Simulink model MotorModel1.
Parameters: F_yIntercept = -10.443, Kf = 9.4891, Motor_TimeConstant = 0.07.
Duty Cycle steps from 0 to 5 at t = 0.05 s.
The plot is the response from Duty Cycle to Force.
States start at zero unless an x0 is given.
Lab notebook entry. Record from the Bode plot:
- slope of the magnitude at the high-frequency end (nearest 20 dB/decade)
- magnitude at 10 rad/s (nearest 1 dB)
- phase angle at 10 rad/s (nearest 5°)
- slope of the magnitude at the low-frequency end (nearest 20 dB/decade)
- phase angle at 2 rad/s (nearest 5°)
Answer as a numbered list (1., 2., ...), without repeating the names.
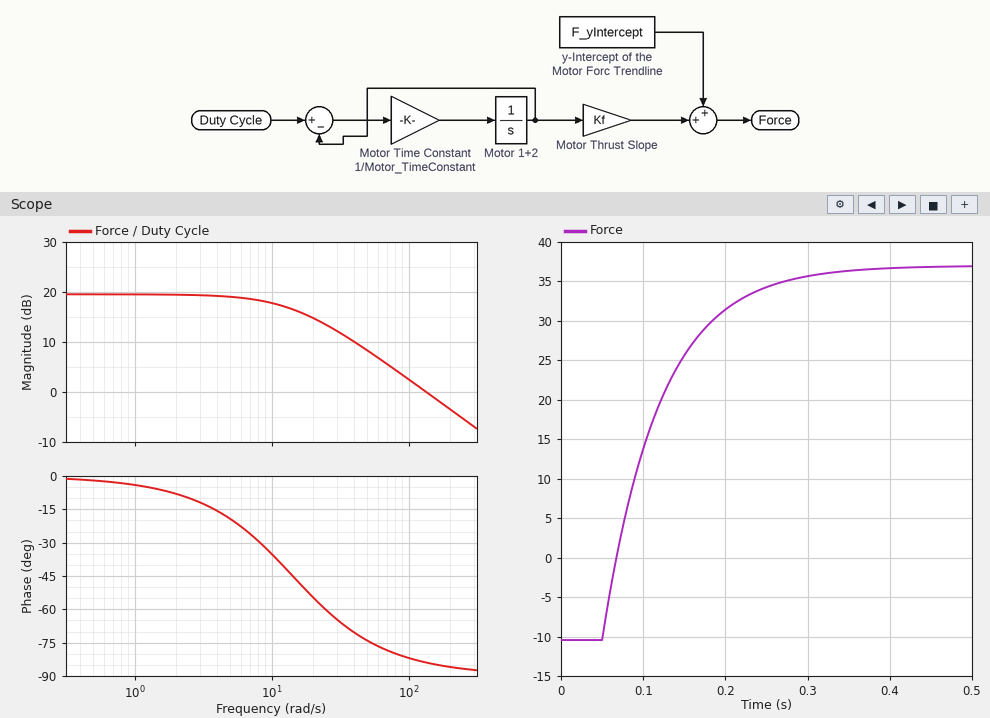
1. -20 dB/decade
2. 18 dB
3. -35°
4. 0 dB/decade
5. -10°
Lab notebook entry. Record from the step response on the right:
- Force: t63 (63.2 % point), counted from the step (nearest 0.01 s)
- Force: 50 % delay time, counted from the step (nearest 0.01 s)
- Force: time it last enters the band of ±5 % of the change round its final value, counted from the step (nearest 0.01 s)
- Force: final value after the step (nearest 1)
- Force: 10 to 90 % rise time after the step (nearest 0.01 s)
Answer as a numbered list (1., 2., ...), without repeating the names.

1. 0.07 s
2. 0.05 s
3. 0.21 s
4. 37
5. 0.15 s
